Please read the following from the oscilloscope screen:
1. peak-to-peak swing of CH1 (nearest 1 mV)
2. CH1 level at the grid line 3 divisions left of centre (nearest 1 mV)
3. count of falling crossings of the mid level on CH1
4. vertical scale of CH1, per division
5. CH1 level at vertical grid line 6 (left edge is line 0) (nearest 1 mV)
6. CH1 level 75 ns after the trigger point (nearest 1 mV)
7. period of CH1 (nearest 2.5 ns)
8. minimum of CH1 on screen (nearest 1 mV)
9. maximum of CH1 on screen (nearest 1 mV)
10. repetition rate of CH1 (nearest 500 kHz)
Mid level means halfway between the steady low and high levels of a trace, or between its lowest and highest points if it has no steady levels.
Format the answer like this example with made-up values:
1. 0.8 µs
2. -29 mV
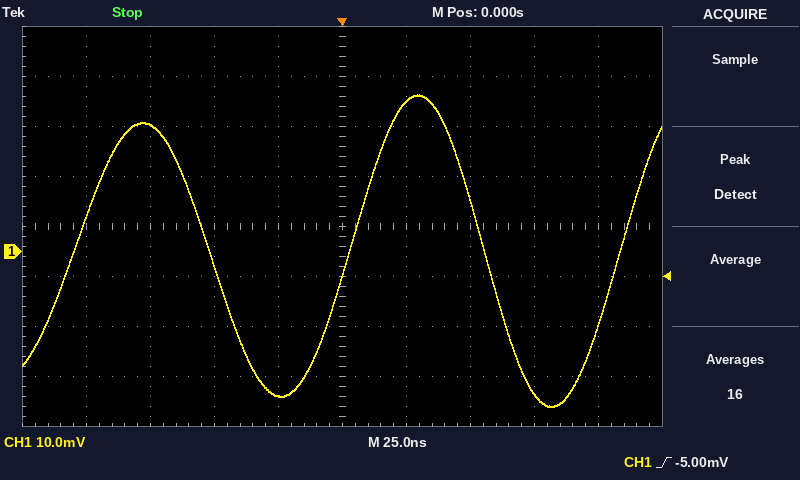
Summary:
1. 62 mV
2. 25 mV
3. 2
4. 10 mV
5. 30 mV
6. -28 mV
7. 107.5 ns
8. -31 mV
9. 31 mV
10. 9.5 MHz
